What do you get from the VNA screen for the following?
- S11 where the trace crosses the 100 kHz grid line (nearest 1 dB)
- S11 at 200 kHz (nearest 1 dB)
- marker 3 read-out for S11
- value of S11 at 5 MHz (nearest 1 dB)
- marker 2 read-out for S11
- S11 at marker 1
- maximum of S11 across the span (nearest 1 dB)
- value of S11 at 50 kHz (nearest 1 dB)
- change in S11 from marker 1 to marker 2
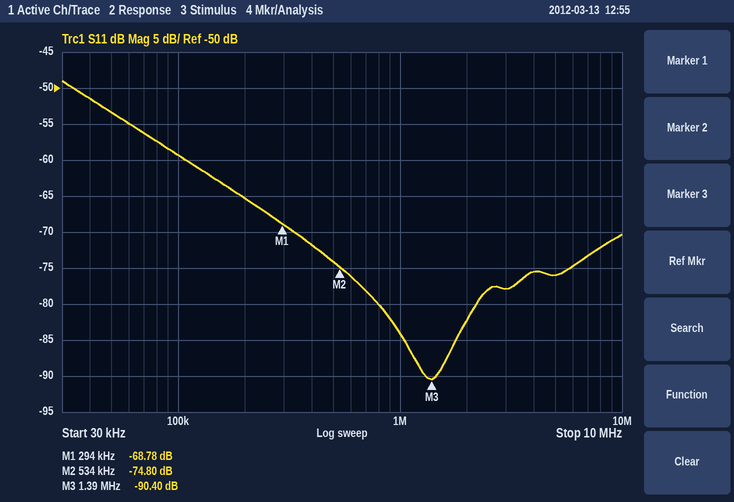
-59 dB
-65 dB
-90.40 dB
-76 dB
-74.80 dB
-68.78 dB
-49 dB
-53 dB
-6.02 dB
